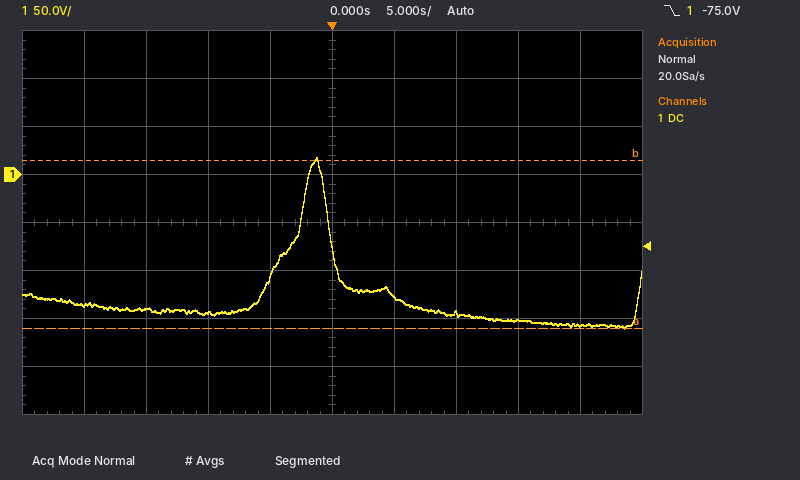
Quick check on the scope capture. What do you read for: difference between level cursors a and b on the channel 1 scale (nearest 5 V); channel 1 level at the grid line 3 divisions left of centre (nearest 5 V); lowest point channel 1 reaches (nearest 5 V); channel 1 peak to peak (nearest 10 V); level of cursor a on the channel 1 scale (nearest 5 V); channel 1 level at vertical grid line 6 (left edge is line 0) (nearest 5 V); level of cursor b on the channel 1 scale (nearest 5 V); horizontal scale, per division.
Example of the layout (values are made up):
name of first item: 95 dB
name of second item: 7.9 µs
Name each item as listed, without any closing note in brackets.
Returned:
difference between level cursors a and b on the channel 1 scale: 175 V
channel 1 level at the grid line 3 divisions left of centre: -140 V
lowest point channel 1 reaches: -160 V
channel 1 peak to peak: 180 V
level of cursor a on the channel 1 scale: -160 V
channel 1 level at vertical grid line 6 (left edge is line 0): -125 V
level of cursor b on the channel 1 scale: 15 V
horizontal scale, per division: 5 s
